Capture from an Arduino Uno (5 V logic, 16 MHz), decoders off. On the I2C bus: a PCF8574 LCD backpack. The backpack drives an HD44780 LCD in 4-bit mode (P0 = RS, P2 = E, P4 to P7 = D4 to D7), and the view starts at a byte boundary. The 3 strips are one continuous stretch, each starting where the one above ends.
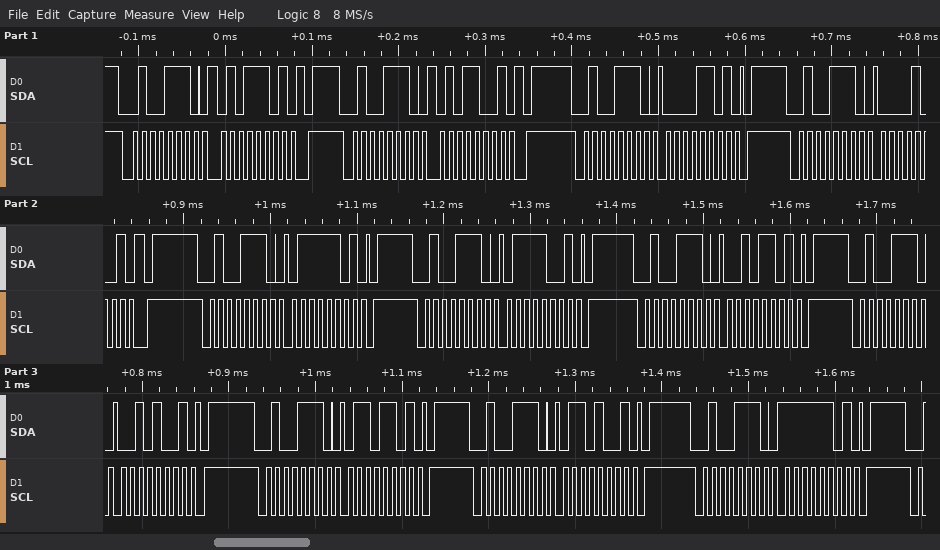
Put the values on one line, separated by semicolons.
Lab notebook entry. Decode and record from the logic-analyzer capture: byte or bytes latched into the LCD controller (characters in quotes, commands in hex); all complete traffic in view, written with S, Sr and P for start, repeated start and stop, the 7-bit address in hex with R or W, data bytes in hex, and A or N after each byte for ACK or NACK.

'P' 'r'; S 27W A 5D A P S 27W A 59 A P S 27W A 0D A P S 27W A 09 A P S 27W A 7D A P S 27W A 79 A P S 27W A 2D A P S 27W A 29 A P S 27W A 6D A P S 27W A 69 A P S 27W A FD A P
